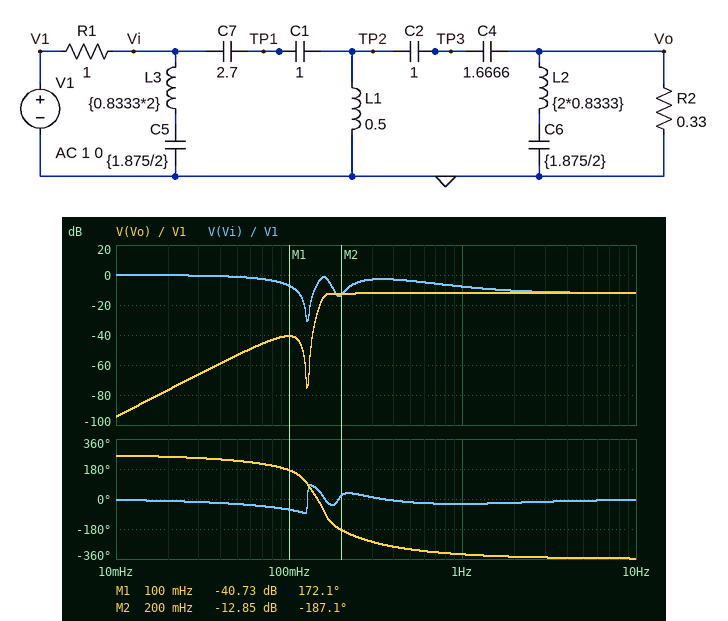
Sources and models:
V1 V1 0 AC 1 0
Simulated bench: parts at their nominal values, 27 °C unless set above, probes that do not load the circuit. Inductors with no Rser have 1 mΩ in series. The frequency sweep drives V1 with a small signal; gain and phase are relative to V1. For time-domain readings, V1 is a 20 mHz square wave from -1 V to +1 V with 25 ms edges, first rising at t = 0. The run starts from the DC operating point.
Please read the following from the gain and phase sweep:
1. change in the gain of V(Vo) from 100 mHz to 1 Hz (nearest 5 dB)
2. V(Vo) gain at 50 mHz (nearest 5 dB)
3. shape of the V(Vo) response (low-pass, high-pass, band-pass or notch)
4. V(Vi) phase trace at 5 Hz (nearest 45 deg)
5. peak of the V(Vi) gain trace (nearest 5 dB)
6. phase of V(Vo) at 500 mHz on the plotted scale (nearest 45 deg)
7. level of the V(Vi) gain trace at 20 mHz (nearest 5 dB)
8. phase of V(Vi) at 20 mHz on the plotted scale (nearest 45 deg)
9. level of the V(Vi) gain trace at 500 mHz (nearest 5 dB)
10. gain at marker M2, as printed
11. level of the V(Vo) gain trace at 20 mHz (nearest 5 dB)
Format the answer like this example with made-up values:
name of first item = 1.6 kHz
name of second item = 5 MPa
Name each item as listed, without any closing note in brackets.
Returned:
change in the gain of V(Vo) from 100 mHz to 1 Hz = 30 dB
V(Vo) gain at 50 mHz = -55 dB
shape of the V(Vo) response = high-pass
V(Vi) phase trace at 5 Hz = 0 deg
peak of the V(Vi) gain trace = 0 dB
phase of V(Vo) at 500 mHz on the plotted scale = -315 deg
level of the V(Vi) gain trace at 20 mHz = 0 dB
phase of V(Vi) at 20 mHz on the plotted scale = 0 deg
level of the V(Vi) gain trace at 500 mHz = -5 dB
gain at marker M2, as printed = -12.85 dB
level of the V(Vo) gain trace at 20 mHz = -75 dB
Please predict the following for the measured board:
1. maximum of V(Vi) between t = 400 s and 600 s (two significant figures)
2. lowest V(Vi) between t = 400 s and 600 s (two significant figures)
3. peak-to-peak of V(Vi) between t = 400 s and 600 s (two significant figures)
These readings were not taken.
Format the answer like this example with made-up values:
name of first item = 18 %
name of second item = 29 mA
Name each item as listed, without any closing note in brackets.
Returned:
maximum of V(Vi) between t = 400 s and 600 s = 1.2 V
lowest V(Vi) between t = 400 s and 600 s = -1.2 V
peak-to-peak of V(Vi) between t = 400 s and 600 s = 2.3 V
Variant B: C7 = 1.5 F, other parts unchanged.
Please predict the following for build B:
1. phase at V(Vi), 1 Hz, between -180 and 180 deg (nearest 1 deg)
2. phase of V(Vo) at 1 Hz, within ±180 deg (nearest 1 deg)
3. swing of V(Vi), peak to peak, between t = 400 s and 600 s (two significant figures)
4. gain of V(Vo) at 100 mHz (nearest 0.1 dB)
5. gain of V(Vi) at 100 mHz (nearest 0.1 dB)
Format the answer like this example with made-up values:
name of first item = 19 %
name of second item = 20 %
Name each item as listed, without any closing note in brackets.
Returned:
phase at V(Vi), 1 Hz, between -180 and 180 deg = -30 deg
phase of V(Vo) at 1 Hz, within ±180 deg = 30 deg
swing of V(Vi), peak to peak, between t = 400 s and 600 s = 2.4 V
gain of V(Vo) at 100 mHz = -42.3 dB
gain of V(Vi) at 100 mHz = -6.9 dB
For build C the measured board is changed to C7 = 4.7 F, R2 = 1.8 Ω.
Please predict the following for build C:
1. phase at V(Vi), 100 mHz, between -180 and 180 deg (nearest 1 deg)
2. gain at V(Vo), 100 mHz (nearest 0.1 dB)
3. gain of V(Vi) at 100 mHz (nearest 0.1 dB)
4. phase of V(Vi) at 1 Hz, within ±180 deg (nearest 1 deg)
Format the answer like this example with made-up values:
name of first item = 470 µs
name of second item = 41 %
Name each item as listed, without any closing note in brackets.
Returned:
phase at V(Vi), 100 mHz, between -180 and 180 deg = -65 deg
gain at V(Vo), 100 mHz = -34.9 dB
gain of V(Vi) at 100 mHz = -7.6 dB
phase of V(Vi) at 1 Hz, within ±180 deg = 13 deg
